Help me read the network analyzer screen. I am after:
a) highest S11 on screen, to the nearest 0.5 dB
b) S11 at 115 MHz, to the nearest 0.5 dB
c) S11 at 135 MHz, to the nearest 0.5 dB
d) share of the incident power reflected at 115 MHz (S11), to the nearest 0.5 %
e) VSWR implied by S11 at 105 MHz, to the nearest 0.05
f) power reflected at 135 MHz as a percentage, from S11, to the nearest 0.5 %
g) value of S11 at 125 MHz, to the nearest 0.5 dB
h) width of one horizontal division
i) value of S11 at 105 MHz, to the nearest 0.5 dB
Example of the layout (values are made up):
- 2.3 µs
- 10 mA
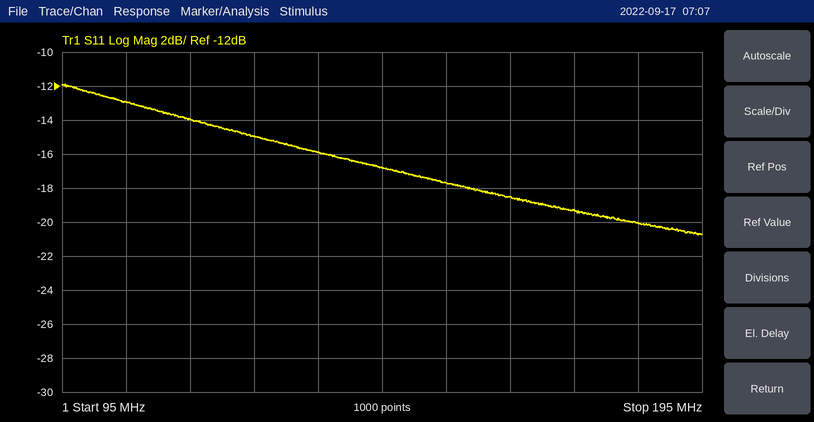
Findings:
- -12.0 dB
- -14.0 dB
- -16.0 dB
- 4.0 %
- 1.60
- 2.5 %
- -15.0 dB
- 10 MHz
- -13.0 dB
